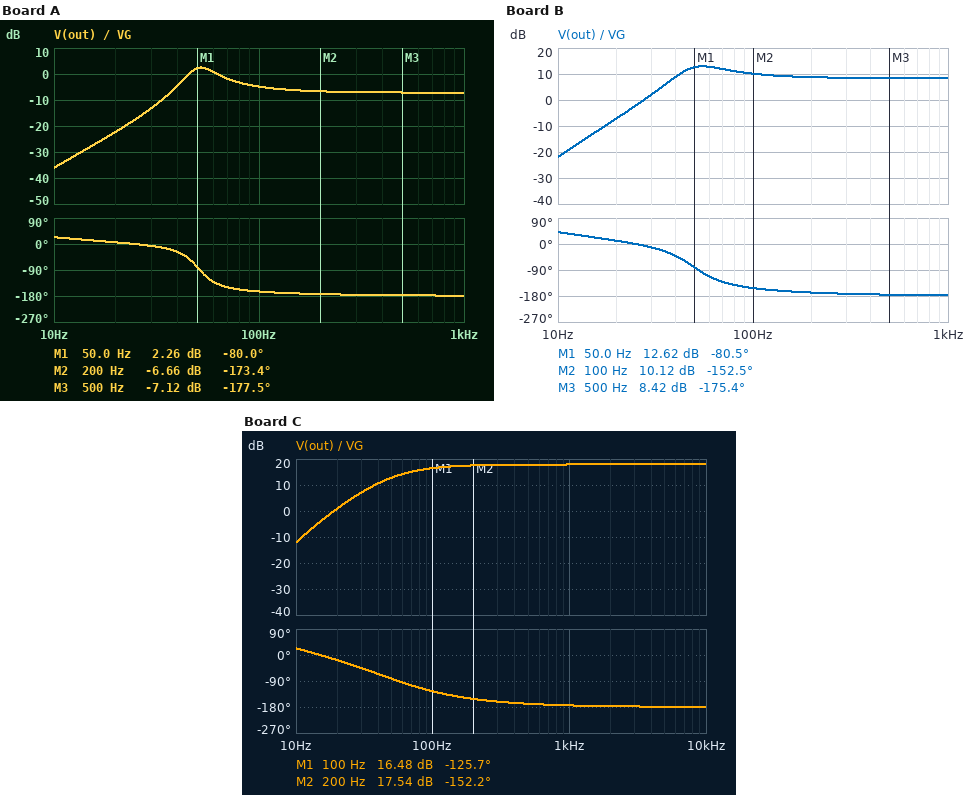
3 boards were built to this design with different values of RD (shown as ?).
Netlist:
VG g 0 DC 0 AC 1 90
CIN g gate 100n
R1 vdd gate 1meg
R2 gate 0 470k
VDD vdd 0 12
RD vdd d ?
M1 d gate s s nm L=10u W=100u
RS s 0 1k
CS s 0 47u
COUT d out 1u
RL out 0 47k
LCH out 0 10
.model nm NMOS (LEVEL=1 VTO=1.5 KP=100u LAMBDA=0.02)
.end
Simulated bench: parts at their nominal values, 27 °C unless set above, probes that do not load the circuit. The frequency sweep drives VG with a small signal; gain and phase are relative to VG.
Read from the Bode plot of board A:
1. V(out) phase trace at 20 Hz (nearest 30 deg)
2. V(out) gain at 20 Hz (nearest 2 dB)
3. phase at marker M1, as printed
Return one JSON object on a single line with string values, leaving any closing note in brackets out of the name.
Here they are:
{"V(out) phase trace at 20 Hz": "0 deg", "V(out) gain at 20 Hz": "-22 dB", "phase at marker M1, as printed": "-80.0 deg"}
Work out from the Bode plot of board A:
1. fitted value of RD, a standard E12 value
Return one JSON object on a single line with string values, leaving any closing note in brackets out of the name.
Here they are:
{"fitted value of RD, a standard E12 value": "15 kΩ"}
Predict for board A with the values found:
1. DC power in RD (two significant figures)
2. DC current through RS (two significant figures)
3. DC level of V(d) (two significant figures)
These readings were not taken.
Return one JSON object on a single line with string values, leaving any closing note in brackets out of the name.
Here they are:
{"DC power in RD": "7.7 mW", "DC current through RS": "720 µA", "DC level of V(d)": "1.2 V"}
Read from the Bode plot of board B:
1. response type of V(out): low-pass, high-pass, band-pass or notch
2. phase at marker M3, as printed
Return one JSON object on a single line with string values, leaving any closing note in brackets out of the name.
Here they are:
{"response type of V(out): low-pass, high-pass, band-pass or notch": "high-pass", "phase at marker M3, as printed": "-175.4 deg"}
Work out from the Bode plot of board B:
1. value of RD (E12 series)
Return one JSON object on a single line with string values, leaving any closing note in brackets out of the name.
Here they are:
{"value of RD": "1.8 kΩ"}
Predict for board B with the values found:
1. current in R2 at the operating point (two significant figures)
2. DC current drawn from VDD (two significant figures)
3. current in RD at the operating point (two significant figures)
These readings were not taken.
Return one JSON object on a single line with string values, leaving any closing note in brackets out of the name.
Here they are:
{"current in R2 at the operating point": "8.2 µA", "DC current drawn from VDD": "1.0 mA", "current in RD at the operating point": "1.0 mA"}
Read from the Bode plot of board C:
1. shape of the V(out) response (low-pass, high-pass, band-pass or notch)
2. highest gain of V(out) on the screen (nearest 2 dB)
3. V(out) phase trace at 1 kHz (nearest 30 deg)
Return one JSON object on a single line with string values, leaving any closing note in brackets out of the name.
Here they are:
{"shape of the V(out) response": "high-pass", "highest gain of V(out) on the screen": "18 dB", "V(out) phase trace at 1 kHz": "-180 deg"}
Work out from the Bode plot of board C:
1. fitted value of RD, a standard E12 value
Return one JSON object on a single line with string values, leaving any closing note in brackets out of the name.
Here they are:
{"fitted value of RD, a standard E12 value": "6.8 kΩ"}
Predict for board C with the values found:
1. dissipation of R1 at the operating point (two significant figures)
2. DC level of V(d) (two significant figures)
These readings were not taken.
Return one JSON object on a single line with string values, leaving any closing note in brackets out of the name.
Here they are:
{"dissipation of R1 at the operating point": "67 µW", "DC level of V(d)": "5.3 V"}
